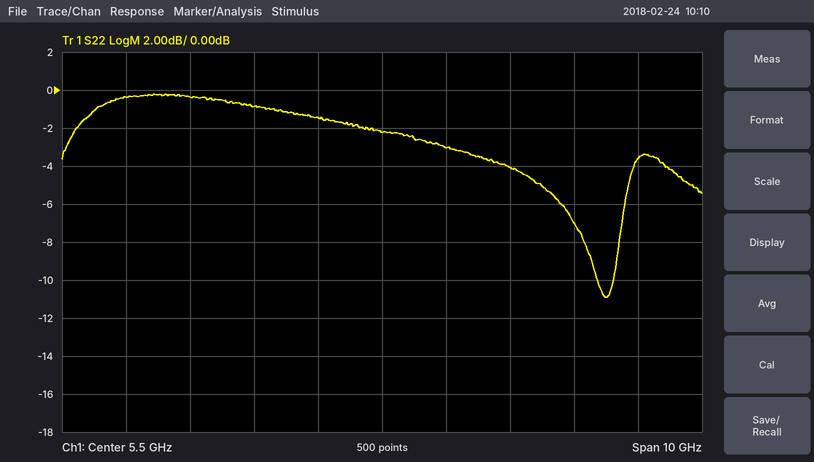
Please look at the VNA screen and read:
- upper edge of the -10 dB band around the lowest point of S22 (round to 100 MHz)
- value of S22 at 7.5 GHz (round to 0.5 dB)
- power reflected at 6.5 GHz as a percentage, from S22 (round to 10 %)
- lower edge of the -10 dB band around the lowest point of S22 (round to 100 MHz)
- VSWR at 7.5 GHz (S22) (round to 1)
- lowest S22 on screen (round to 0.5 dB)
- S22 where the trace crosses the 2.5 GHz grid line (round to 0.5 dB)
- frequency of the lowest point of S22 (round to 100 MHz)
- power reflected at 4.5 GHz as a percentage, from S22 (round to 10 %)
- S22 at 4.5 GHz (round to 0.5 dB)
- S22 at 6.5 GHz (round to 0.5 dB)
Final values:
9.1 GHz
-4.0 dB
50 %
8.9 GHz
4
-11.0 dB
-0.5 dB
9.0 GHz
70 %
-1.5 dB
-3.0 dB
